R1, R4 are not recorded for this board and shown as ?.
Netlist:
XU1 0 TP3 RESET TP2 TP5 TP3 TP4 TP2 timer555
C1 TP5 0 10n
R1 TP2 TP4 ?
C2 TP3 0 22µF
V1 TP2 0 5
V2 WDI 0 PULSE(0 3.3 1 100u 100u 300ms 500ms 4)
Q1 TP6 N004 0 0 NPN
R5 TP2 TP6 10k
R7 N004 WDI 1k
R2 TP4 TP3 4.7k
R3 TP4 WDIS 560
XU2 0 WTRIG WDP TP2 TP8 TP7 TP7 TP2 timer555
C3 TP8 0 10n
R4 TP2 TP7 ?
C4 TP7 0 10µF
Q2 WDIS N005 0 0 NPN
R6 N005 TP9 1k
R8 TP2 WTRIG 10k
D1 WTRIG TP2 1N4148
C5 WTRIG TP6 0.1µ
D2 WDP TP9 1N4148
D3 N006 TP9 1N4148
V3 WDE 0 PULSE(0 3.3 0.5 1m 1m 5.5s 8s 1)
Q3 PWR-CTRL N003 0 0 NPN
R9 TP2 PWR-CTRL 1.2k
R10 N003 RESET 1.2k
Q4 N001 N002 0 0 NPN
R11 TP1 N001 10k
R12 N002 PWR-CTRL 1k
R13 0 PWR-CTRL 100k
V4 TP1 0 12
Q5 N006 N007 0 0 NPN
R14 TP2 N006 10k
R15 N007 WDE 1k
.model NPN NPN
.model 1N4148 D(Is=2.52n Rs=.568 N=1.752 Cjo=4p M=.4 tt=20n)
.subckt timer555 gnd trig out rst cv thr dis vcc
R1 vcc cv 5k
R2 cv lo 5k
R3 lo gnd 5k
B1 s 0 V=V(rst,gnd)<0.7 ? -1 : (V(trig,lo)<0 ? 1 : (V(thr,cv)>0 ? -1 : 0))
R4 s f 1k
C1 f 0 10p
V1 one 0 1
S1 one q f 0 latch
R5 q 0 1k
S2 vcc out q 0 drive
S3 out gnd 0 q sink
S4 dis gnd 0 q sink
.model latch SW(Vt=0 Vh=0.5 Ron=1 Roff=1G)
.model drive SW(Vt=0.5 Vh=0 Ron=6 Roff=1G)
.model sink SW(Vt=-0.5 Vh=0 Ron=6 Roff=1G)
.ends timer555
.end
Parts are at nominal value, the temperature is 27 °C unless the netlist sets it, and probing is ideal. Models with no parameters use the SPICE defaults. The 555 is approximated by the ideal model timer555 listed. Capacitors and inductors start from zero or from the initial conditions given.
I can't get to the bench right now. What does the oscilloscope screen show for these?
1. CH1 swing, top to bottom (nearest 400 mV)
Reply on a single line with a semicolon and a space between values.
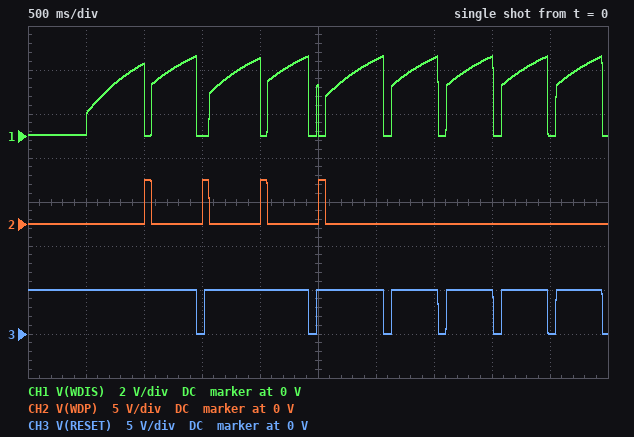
3.6 V
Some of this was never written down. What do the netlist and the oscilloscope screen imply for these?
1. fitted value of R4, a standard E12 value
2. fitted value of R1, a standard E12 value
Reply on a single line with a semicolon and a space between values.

5.6 kΩ; 22 kΩ
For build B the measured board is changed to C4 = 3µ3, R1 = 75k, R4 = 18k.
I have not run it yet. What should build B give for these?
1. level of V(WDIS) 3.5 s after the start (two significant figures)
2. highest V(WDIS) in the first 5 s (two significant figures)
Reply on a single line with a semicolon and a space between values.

2.9 V; 3.4 V
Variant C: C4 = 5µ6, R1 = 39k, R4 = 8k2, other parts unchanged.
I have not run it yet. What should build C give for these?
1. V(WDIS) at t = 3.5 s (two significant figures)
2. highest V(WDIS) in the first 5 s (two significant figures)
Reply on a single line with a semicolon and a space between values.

2.9 V; 3.5 V
